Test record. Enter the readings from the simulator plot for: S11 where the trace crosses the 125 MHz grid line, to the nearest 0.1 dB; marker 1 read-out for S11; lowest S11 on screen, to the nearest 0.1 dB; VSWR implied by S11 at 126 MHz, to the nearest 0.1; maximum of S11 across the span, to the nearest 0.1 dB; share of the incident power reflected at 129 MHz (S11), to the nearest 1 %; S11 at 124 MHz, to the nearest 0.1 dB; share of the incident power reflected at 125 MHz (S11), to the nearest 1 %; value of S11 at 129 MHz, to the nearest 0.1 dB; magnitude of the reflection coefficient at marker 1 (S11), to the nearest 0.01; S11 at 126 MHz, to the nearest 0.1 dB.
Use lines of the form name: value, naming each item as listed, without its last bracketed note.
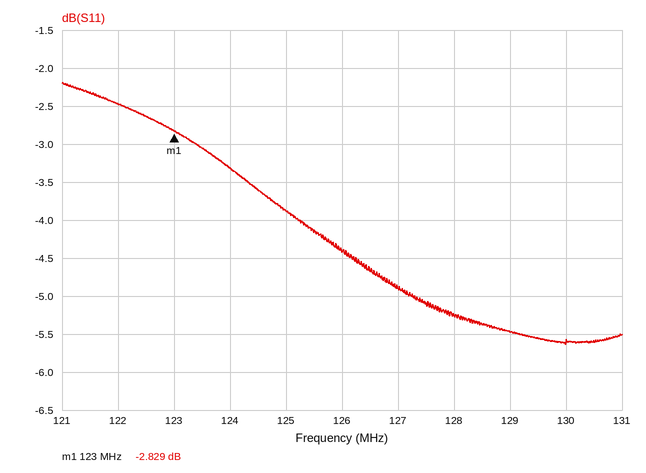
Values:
S11 where the trace crosses the 125 MHz grid line, to the nearest 0.1 dB: -3.9 dB
marker 1 read-out for S11: -2.829 dB
lowest S11 on screen, to the nearest 0.1 dB: -5.6 dB
VSWR implied by S11 at 126 MHz, to the nearest 0.1: 4.0
maximum of S11 across the span, to the nearest 0.1 dB: -2.2 dB
share of the incident power reflected at 129 MHz (S11), to the nearest 1 %: 28 %
S11 at 124 MHz, to the nearest 0.1 dB: -3.3 dB
share of the incident power reflected at 125 MHz (S11), to the nearest 1 %: 41 %
value of S11 at 129 MHz, to the nearest 0.1 dB: -5.5 dB
magnitude of the reflection coefficient at marker 1 (S11), to the nearest 0.01: 0.72
S11 at 126 MHz, to the nearest 0.1 dB: -4.4 dB
